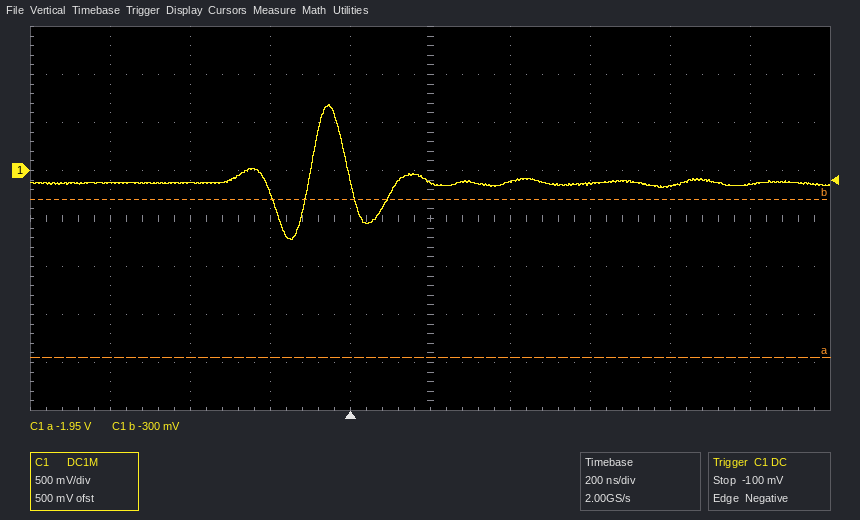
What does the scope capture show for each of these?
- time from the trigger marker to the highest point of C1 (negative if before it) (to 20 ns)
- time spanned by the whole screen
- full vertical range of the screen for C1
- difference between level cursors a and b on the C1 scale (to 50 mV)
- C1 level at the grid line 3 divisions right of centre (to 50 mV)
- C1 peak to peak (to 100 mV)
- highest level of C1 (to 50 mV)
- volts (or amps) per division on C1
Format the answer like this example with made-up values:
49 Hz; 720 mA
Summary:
-60 ns; 2 µs; 4 V; 1.65 V; -150 mV; 1.40 V; 700 mV; 500 mV
